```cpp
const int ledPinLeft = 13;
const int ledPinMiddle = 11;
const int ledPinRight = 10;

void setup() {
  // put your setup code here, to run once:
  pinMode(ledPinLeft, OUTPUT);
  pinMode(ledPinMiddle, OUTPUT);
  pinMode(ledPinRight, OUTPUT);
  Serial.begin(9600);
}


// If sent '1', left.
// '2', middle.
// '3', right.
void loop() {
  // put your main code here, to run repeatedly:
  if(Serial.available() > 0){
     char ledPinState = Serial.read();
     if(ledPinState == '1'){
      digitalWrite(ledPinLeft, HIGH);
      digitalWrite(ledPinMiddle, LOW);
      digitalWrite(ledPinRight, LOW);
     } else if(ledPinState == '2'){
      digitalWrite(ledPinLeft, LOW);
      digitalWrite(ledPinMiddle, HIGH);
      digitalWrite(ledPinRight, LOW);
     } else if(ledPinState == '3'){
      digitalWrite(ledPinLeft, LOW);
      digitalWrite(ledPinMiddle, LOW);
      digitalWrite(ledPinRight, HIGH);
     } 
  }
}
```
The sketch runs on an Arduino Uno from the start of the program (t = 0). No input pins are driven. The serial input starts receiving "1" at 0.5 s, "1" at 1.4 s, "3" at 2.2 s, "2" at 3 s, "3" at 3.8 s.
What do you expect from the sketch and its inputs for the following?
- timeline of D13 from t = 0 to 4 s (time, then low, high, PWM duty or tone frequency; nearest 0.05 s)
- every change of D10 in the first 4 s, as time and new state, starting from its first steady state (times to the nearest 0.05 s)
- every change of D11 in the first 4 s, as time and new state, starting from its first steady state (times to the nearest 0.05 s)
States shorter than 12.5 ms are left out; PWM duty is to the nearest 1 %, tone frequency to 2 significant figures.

0 s low; 0.5 s high; 2.2 s low
0 s low; 2.2 s high; 3 s low; 3.8 s high
0 s low; 3 s high; 3.8 s low
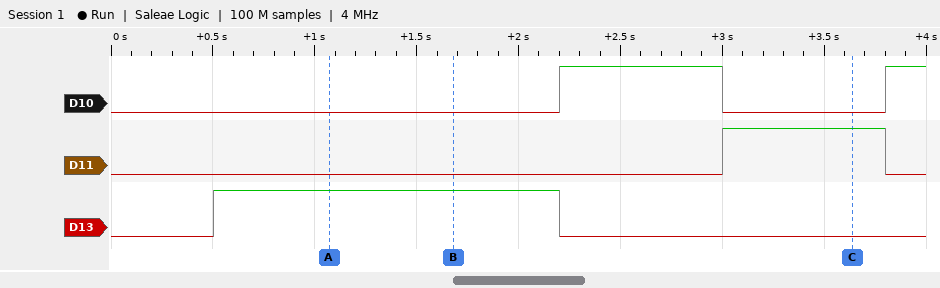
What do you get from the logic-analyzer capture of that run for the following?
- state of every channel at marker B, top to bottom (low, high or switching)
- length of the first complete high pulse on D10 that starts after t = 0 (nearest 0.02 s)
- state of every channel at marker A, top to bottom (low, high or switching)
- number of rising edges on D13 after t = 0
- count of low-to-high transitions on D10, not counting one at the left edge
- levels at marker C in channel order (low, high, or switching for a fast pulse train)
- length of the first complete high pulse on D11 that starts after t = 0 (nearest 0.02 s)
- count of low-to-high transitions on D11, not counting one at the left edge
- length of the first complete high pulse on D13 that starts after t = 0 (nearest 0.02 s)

D10 low, D11 low, D13 high
0.80 s
D10 low, D11 low, D13 high
1
2
D10 low, D11 high, D13 low
0.80 s
1
1.70 s
